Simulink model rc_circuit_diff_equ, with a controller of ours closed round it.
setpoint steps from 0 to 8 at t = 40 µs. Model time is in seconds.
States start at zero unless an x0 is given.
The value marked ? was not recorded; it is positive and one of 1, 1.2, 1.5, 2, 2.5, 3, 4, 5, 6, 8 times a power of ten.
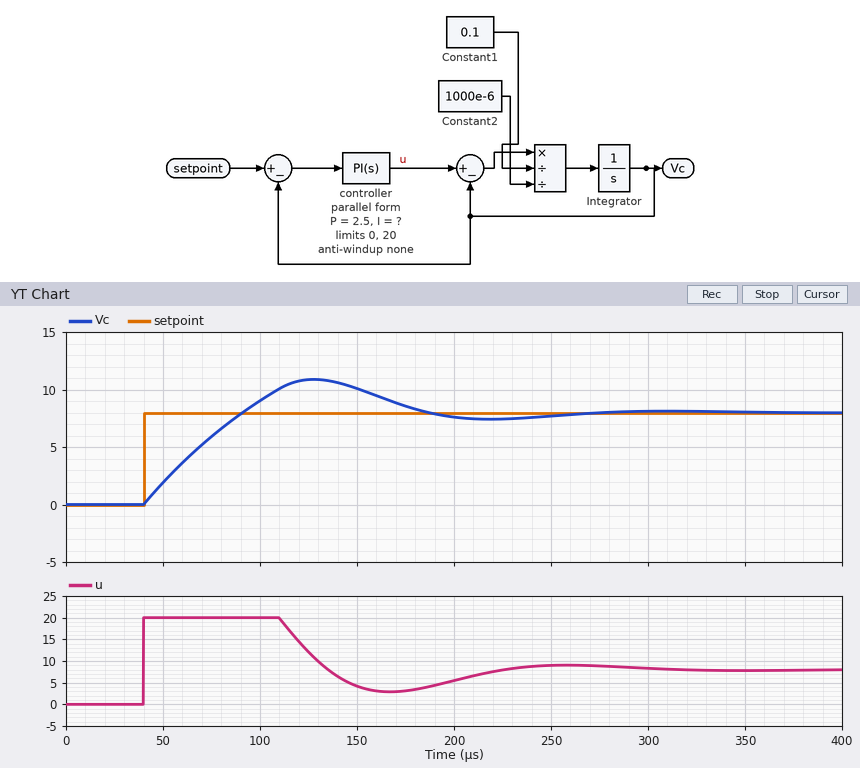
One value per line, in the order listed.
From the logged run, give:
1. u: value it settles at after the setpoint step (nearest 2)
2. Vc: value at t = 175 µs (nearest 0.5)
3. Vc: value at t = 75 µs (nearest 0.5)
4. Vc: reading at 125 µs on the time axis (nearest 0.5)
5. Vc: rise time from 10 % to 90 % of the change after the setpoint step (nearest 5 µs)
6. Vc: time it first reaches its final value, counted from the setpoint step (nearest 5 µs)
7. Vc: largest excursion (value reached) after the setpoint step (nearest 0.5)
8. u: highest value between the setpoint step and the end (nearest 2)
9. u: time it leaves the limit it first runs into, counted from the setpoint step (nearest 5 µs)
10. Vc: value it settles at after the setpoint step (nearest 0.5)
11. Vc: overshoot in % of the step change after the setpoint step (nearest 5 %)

8
8.5
6.0
11.0
40 µs
50 µs
11.0
20
70 µs
8.0
35 %
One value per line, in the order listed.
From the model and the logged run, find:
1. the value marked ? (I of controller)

150000
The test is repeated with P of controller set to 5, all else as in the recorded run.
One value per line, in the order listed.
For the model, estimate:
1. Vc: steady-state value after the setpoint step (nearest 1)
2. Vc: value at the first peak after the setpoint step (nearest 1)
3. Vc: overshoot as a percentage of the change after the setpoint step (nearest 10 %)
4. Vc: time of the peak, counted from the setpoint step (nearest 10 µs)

8
10
30 %
80 µs
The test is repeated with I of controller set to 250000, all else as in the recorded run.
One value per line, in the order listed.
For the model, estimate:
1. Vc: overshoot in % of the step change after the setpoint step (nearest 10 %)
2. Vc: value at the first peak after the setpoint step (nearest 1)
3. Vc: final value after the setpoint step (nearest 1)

50 %
12
8
